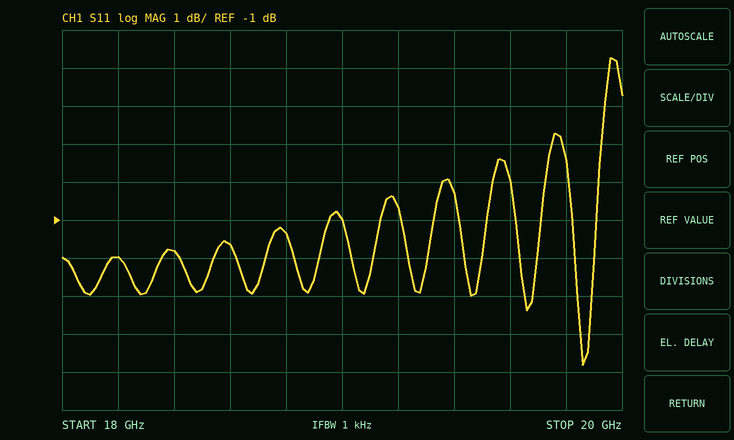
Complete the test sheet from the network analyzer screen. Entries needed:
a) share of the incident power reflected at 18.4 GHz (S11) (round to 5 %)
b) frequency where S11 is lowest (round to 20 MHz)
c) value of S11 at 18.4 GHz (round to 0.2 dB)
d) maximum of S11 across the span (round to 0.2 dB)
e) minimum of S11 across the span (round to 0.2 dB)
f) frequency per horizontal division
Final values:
65 %
19.86 GHz
-1.8 dB
3.2 dB
-4.8 dB
200 MHz
